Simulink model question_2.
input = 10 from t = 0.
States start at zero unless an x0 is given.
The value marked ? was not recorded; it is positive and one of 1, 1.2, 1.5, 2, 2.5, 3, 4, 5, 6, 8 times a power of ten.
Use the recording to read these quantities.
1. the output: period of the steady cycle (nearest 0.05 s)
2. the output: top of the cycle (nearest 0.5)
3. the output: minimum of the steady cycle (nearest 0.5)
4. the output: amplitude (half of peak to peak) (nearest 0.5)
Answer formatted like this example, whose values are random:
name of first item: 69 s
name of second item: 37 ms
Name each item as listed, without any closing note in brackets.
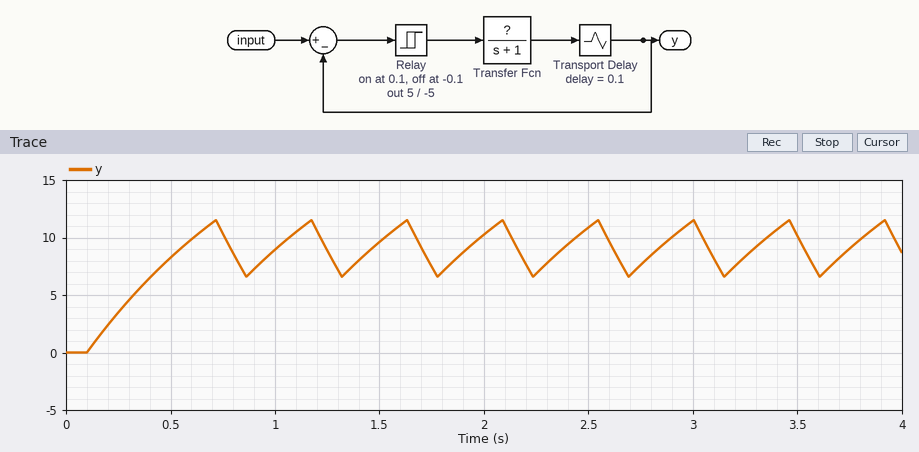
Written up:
the output: period of the steady cycle: 0.45 s
the output: top of the cycle: 11.5
the output: minimum of the steady cycle: 6.5
the output: amplitude (half of peak to peak): 2.5
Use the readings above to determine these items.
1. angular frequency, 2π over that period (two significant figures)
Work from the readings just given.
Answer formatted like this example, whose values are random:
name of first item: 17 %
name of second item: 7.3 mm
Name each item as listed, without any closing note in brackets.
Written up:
angular frequency, 2π over that period: 14 rad/s
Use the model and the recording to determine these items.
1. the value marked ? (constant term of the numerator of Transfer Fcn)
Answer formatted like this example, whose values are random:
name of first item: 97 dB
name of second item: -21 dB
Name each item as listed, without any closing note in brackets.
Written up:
the value marked ?: 5
